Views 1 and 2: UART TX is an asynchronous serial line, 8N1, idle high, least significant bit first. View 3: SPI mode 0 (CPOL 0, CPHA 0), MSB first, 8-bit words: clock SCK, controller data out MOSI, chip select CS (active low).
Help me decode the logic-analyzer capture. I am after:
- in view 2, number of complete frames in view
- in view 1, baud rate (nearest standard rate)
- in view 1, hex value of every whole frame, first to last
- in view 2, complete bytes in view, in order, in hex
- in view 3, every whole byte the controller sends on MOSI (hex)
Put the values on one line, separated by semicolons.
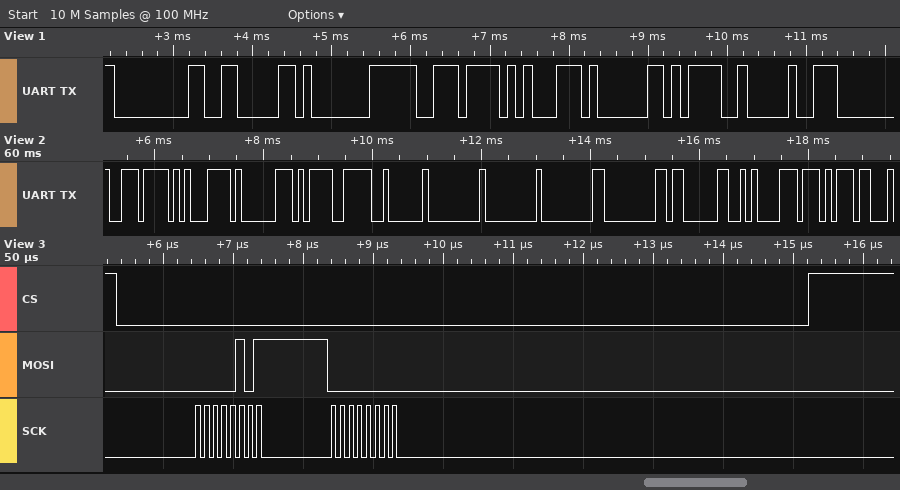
12; 9600 baud; 00 06 01 EE C5 81 3D 90; EE C5 81 3D 02 00 00 00 00 03 0A D7; 0x05 0x00
